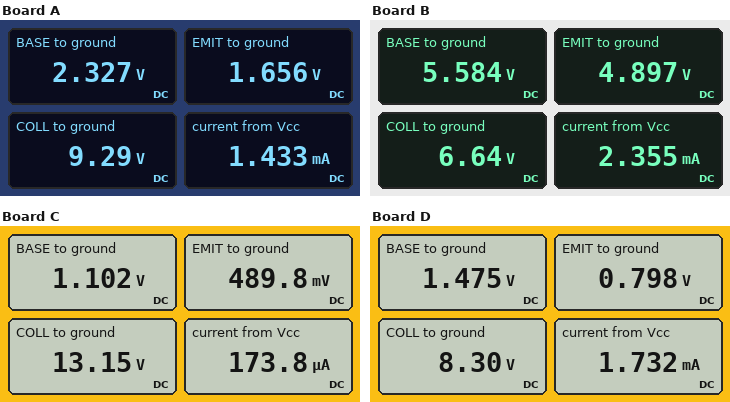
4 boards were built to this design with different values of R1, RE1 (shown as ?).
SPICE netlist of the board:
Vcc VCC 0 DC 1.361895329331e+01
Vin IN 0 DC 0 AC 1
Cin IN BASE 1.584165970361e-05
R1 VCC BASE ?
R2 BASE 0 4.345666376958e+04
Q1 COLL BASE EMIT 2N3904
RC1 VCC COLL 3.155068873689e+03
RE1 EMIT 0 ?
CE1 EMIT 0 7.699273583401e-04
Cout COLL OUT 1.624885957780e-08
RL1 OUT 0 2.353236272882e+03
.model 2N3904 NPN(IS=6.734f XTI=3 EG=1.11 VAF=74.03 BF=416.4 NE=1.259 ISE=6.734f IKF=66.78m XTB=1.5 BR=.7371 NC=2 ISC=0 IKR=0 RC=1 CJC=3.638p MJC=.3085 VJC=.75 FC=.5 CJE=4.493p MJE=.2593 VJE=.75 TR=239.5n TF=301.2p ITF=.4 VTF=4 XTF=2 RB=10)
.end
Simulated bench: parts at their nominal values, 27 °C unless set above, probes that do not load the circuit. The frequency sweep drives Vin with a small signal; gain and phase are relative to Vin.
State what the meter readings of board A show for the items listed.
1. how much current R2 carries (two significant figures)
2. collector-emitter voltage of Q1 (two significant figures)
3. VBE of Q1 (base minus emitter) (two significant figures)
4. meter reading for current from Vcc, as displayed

54 µA
7.6 V
670 mV
1.433 mA
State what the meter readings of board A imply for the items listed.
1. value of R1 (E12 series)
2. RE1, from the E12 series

180 kΩ
1.2 kΩ
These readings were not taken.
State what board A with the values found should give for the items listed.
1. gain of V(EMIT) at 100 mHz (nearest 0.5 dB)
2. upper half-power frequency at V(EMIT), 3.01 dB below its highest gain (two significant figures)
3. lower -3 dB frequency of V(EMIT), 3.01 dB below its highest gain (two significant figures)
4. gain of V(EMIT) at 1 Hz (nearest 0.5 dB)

-11.5 dB
14 Hz
250 mHz
-2.5 dB
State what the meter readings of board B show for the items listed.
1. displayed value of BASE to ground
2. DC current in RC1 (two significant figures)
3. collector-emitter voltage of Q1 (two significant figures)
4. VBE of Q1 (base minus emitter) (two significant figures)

5.584 V
2.2 mA
1.7 V
690 mV
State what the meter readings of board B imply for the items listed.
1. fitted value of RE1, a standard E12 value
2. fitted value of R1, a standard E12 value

2.2 kΩ
56 kΩ
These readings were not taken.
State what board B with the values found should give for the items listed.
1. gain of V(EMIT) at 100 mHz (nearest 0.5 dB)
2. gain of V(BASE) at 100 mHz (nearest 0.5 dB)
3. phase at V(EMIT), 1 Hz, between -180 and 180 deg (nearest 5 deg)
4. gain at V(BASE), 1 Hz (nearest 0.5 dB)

-13.5 dB
-13.5 dB
15 deg
-3.0 dB
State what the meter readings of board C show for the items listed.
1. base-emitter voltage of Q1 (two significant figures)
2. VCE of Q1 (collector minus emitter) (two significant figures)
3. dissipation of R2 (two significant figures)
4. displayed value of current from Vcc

610 mV
13 V
28 µW
173.8 µA
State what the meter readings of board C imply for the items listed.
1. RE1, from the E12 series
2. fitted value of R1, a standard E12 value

3.3 kΩ
470 kΩ
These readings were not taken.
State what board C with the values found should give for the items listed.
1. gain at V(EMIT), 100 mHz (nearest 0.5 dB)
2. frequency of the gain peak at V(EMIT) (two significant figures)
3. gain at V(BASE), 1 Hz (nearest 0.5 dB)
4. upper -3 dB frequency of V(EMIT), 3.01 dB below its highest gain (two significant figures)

-10.0 dB
580 mHz
-2.0 dB
2.1 Hz
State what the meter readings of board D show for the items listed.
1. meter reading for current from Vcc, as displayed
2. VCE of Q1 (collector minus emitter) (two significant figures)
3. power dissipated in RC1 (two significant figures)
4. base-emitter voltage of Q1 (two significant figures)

1.732 mA
7.5 V
9.0 mW
680 mV
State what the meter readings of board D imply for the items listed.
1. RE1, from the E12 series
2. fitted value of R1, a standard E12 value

470 Ω
270 kΩ
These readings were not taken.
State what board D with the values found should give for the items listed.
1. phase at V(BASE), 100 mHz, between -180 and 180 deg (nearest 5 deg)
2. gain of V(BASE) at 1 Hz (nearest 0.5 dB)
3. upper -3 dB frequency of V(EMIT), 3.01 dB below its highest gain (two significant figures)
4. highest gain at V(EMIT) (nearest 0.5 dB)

70 deg
-2.5 dB
17 Hz
-2.5 dB
